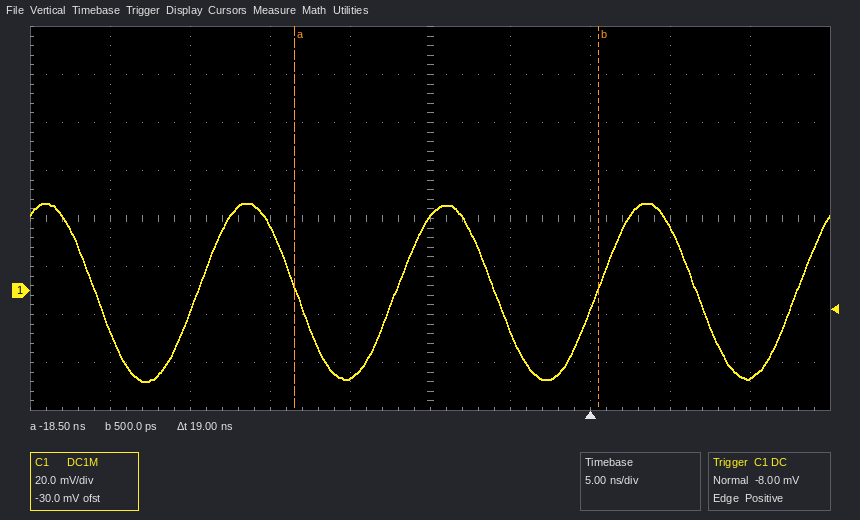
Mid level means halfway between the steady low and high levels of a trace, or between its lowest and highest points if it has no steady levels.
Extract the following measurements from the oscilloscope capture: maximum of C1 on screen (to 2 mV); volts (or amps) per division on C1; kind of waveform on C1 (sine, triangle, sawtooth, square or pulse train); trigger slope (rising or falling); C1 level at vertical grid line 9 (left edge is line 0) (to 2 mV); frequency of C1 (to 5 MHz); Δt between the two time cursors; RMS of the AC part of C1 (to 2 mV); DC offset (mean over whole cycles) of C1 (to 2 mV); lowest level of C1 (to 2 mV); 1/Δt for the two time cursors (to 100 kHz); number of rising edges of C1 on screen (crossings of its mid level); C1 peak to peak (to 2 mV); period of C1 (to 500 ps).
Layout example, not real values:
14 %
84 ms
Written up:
36 mV
20 mV
sine
rising
-36 mV
80 MHz
19 ns
26 mV
0 mV
-38 mV
52.6 MHz
4
74 mV
12.5 ns
